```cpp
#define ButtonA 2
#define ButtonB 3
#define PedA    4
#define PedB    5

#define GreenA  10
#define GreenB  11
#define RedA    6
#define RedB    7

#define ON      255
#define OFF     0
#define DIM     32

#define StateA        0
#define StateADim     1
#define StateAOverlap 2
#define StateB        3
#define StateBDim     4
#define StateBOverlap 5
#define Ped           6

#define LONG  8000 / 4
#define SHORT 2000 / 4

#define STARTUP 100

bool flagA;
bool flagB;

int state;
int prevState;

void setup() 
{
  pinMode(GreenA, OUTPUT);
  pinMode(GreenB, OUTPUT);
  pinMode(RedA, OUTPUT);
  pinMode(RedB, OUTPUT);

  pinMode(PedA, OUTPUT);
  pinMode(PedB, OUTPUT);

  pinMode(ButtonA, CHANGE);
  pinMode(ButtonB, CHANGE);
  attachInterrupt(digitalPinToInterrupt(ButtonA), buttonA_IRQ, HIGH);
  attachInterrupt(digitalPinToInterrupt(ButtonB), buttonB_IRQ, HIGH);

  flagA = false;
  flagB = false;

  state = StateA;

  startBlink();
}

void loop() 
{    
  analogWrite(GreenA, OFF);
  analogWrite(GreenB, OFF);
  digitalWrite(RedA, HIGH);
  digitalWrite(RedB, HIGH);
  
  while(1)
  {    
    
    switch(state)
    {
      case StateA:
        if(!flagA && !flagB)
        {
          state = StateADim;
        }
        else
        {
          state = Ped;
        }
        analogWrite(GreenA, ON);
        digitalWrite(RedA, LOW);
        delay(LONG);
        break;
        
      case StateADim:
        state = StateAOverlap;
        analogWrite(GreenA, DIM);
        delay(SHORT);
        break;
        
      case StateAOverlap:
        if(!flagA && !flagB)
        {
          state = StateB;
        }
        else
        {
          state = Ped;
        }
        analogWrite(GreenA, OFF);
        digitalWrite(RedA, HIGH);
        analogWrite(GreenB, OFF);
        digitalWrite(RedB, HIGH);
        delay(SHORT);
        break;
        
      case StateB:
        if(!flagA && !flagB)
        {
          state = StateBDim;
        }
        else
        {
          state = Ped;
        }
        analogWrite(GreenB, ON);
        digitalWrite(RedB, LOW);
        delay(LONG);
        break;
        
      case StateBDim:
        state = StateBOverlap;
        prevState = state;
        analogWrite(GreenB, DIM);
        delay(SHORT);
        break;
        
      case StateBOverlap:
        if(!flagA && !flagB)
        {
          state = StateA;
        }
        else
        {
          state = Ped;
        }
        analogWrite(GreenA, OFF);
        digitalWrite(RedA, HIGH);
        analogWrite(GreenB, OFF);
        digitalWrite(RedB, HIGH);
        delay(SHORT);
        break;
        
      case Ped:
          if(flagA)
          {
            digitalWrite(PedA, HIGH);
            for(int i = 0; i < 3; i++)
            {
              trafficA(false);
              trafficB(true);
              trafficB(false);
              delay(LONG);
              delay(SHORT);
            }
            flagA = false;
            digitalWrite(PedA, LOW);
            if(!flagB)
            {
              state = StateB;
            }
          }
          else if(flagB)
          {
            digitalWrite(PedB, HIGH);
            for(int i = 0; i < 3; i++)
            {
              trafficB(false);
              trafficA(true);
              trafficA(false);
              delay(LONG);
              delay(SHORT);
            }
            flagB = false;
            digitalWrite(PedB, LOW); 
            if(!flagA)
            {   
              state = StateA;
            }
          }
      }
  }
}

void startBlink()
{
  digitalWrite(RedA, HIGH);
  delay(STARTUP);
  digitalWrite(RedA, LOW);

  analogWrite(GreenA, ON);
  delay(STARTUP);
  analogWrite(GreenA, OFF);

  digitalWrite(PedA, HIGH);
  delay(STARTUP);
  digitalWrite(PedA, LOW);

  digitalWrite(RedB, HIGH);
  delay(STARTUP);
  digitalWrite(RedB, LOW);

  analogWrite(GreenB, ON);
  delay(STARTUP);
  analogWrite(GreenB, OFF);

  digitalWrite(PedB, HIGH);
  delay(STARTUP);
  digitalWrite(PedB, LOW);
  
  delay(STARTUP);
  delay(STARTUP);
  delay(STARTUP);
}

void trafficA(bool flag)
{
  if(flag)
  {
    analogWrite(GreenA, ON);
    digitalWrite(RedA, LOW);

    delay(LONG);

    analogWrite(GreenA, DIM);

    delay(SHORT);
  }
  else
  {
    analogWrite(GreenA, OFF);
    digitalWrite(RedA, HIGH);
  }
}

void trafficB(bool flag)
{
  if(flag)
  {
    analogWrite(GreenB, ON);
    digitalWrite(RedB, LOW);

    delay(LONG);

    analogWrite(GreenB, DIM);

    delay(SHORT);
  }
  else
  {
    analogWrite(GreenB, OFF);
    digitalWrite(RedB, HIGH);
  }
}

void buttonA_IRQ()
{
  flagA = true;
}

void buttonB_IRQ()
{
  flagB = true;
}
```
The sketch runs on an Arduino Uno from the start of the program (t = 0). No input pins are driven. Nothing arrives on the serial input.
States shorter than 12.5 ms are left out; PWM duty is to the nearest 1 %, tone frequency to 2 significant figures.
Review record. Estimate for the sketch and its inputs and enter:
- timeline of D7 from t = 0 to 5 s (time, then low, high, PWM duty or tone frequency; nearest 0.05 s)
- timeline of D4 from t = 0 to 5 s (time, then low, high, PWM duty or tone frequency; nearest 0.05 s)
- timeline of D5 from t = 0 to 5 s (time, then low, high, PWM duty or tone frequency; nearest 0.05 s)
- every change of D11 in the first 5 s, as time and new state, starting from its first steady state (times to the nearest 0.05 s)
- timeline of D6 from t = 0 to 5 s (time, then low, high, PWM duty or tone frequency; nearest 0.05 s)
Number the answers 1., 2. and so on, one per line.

1. 0 s low; 0.3 s high; 0.4 s low; 0.9 s high; 3.9 s low
2. 0 s low; 0.2 s high; 0.3 s low
3. 0 s low; 0.5 s high; 0.6 s low
4. 0 s low; 0.4 s high; 0.5 s low; 3.9 s high
5. 0 s high; 0.1 s low; 3.4 s high
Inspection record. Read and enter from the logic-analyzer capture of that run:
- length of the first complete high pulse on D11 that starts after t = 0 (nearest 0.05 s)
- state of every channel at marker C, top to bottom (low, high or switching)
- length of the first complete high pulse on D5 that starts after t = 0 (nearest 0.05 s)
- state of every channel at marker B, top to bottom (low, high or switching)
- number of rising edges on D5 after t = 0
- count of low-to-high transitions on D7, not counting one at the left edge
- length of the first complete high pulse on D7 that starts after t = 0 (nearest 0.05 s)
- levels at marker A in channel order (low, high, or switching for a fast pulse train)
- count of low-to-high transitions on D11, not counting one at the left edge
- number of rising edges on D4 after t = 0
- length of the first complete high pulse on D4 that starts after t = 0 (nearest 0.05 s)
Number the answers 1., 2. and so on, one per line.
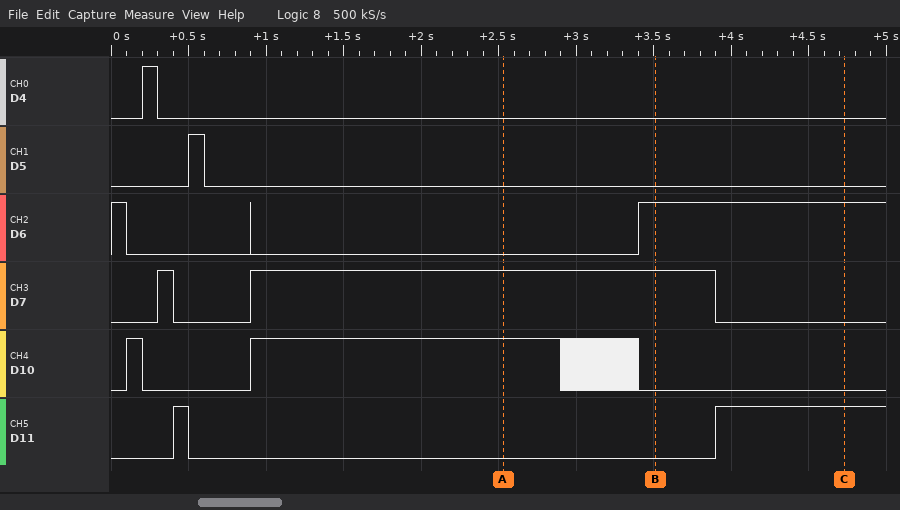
1. 0.10 s
2. D4 low, D5 low, D6 high, D7 low, D10 low, D11 high
3. 0.10 s
4. D4 low, D5 low, D6 high, D7 high, D10 low, D11 low
5. 1
6. 2
7. 0.10 s
8. D4 low, D5 low, D6 low, D7 high, D10 high, D11 low
9. 2
10. 1
11. 0.10 s
